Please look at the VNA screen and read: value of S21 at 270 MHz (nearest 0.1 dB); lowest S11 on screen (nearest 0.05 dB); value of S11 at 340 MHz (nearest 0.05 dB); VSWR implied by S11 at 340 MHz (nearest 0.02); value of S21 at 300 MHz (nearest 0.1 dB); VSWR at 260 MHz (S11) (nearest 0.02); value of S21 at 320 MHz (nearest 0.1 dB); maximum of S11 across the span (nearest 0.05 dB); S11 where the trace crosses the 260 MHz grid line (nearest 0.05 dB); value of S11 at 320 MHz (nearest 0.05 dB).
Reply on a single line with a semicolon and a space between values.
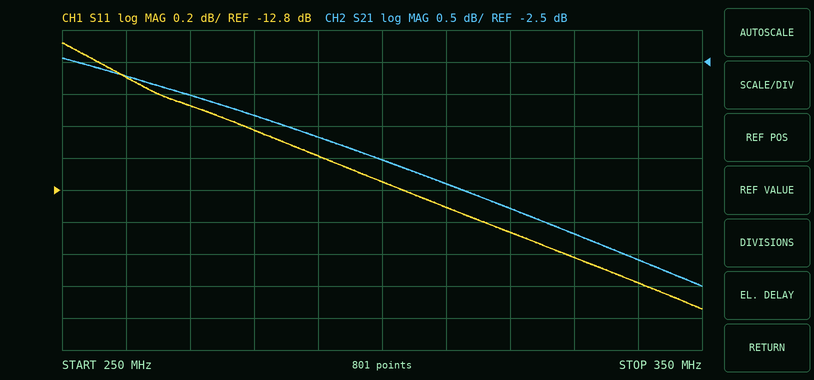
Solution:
-3.0 dB; -13.55 dB; -13.40 dB; 1.54; -4.0 dB; 1.66; -4.8 dB; -11.90 dB; -12.10 dB; -13.05 dB
